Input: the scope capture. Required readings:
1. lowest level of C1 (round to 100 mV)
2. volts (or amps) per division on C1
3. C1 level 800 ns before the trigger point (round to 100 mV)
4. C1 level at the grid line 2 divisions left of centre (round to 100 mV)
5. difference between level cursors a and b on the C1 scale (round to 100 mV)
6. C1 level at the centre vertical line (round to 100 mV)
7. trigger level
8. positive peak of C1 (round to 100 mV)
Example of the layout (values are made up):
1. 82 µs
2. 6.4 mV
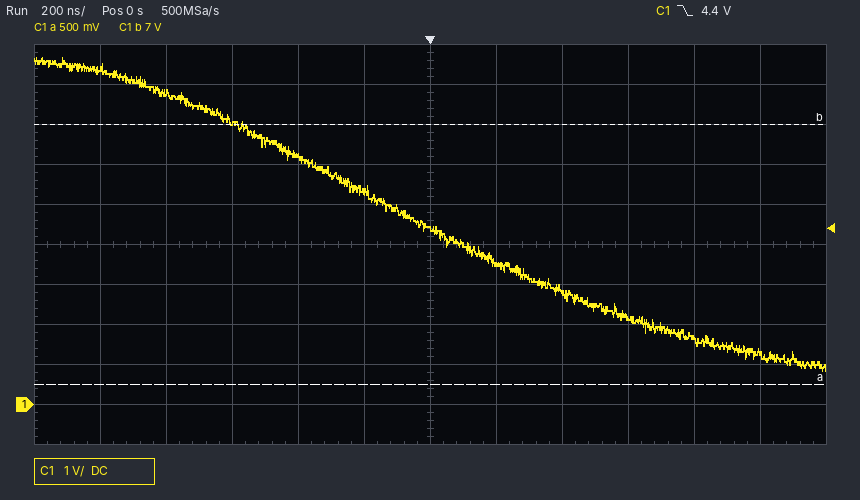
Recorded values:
1. 800 mV
2. 1 V
3. 7.8 V
4. 6.2 V
5. 6.5 V
6. 4.4 V
7. 4.4 V
8. 8.7 V
